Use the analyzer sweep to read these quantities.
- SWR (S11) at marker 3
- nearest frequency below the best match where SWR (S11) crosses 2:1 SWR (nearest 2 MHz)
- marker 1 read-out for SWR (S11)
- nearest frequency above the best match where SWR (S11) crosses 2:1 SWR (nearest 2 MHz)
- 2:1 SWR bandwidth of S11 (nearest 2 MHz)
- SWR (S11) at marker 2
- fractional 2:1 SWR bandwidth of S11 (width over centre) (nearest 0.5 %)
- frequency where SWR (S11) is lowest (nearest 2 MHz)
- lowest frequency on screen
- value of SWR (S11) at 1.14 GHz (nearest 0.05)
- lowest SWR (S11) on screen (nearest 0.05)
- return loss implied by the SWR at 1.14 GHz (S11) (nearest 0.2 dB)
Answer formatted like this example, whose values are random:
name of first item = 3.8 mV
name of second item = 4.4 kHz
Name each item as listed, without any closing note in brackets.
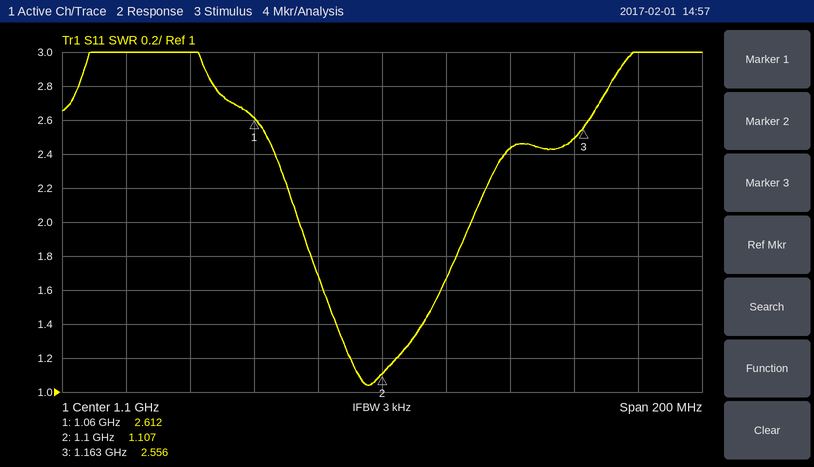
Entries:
SWR (S11) at marker 3 = 2.556
nearest frequency below the best match where SWR (S11) crosses 2:1 SWR = 1.074 GHz
marker 1 read-out for SWR = 2.612
nearest frequency above the best match where SWR (S11) crosses 2:1 SWR = 1.128 GHz
2:1 SWR bandwidth of S11 = 54 MHz
SWR (S11) at marker 2 = 1.107
fractional 2:1 SWR bandwidth of S11 (width over centre) = 5.0 %
frequency where SWR (S11) is lowest = 1.096 GHz
lowest frequency on screen = 1 GHz
value of SWR (S11) at 1.14 GHz = 2.45
lowest SWR (S11) on screen = 1.05
return loss implied by the SWR at 1.14 GHz (S11) = 7.6 dB
